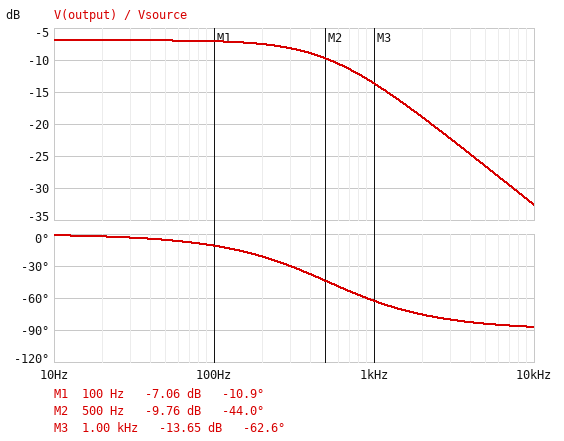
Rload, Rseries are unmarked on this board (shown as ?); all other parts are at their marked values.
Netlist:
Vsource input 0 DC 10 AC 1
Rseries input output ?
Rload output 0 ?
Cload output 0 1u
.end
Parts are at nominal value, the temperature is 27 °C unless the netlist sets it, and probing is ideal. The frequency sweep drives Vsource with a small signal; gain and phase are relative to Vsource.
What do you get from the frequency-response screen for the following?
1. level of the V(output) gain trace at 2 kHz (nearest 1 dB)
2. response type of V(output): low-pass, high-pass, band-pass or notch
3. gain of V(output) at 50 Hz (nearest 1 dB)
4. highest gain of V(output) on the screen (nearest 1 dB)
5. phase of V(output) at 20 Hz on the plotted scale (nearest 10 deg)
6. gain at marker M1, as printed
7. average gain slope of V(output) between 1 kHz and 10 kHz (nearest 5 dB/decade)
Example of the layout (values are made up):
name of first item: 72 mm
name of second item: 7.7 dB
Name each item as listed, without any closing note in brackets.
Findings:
level of the V(output) gain trace at 2 kHz: -19 dB
response type of V(output): low-pass, high-pass, band-pass or notch: low-pass
gain of V(output) at 50 Hz: -7 dB
highest gain of V(output) on the screen: -7 dB
phase of V(output) at 20 Hz on the plotted scale: 0 deg
gain at marker M1, as printed: -7.06 dB
average gain slope of V(output) between 1 kHz and 10 kHz: -20 dB/decade
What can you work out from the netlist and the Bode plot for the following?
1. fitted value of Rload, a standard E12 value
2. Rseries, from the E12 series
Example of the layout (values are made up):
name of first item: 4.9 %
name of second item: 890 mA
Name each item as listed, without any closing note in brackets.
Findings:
fitted value of Rload, a standard E12 value: 560 Ω
Rseries, from the E12 series: 680 Ω
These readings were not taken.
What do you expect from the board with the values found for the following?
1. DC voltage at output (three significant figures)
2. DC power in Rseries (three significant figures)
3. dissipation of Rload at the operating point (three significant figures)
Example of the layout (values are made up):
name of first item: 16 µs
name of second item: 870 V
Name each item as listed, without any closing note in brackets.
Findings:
DC voltage at output: 4.52 V
DC power in Rseries: 44.2 mW
dissipation of Rload at the operating point: 36.4 mW
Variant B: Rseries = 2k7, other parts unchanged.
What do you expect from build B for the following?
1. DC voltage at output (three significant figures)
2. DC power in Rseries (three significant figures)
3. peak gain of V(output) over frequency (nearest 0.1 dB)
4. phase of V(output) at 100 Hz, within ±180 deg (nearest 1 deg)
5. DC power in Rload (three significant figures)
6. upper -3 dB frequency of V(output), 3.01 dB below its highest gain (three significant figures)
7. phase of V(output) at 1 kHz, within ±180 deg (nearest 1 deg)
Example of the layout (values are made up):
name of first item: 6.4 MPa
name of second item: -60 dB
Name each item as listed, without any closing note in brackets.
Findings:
DC voltage at output: 1.72 V
DC power in Rseries: 25.4 mW
peak gain of V(output) over frequency: -15.3 dB
phase of V(output) at 100 Hz, within ±180 deg: -16 deg
DC power in Rload: 5.27 mW
upper -3 dB frequency of V(output), 3.01 dB below its highest gain: 343 Hz
phase of V(output) at 1 kHz, within ±180 deg: -71 deg
